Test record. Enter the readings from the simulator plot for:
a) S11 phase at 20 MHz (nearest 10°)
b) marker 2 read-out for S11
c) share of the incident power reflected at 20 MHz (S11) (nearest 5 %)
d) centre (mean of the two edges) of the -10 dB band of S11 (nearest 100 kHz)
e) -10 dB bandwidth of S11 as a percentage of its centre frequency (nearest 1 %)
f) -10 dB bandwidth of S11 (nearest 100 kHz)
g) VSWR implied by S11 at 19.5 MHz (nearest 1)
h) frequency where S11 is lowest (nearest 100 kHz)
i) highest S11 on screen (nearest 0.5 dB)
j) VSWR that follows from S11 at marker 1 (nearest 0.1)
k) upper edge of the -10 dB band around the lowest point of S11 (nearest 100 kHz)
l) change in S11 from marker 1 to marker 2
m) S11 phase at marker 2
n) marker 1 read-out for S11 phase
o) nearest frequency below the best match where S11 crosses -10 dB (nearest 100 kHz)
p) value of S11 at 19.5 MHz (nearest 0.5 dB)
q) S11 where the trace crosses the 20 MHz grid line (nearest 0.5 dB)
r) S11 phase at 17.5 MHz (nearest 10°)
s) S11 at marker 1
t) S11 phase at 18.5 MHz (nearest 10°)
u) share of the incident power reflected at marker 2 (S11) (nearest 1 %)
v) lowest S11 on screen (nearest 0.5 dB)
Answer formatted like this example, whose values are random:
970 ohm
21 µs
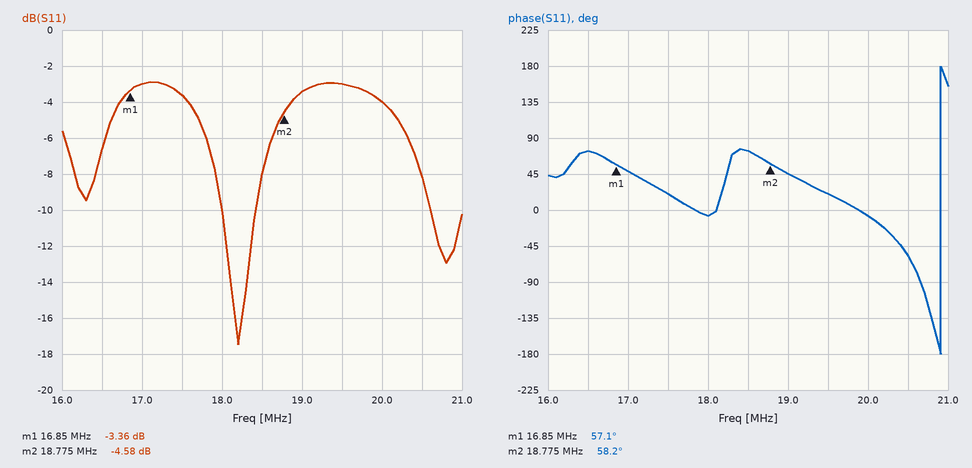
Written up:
-10°
-4.58 dB
40 %
18.2 MHz
2 %
400 kHz
6
18.2 MHz
-3.0 dB
5.2
18.4 MHz
-1.22 dB
58.2°
57.1°
18.0 MHz
-3.0 dB
-4.0 dB
20°
-3.36 dB
70°
35 %
-17.5 dB
